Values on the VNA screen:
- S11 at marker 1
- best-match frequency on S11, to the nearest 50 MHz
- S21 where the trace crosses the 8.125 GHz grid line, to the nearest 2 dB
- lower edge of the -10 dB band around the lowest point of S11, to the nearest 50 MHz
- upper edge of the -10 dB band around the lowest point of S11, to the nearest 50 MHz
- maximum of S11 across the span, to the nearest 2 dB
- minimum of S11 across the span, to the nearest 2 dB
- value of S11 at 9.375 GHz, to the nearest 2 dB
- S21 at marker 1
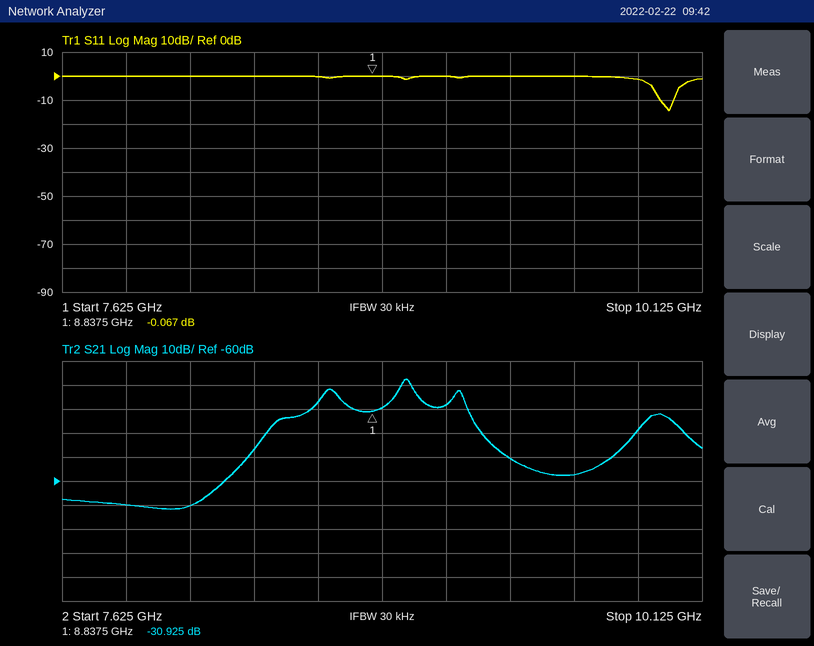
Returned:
-0.067 dB
10.00 GHz
-70 dB
9.95 GHz
10.00 GHz
0 dB
-14 dB
0 dB
-30.925 dB
